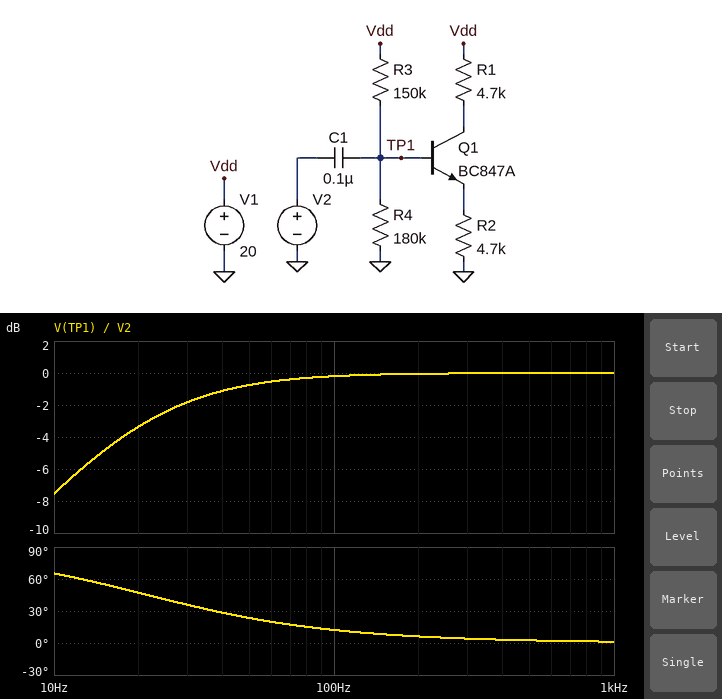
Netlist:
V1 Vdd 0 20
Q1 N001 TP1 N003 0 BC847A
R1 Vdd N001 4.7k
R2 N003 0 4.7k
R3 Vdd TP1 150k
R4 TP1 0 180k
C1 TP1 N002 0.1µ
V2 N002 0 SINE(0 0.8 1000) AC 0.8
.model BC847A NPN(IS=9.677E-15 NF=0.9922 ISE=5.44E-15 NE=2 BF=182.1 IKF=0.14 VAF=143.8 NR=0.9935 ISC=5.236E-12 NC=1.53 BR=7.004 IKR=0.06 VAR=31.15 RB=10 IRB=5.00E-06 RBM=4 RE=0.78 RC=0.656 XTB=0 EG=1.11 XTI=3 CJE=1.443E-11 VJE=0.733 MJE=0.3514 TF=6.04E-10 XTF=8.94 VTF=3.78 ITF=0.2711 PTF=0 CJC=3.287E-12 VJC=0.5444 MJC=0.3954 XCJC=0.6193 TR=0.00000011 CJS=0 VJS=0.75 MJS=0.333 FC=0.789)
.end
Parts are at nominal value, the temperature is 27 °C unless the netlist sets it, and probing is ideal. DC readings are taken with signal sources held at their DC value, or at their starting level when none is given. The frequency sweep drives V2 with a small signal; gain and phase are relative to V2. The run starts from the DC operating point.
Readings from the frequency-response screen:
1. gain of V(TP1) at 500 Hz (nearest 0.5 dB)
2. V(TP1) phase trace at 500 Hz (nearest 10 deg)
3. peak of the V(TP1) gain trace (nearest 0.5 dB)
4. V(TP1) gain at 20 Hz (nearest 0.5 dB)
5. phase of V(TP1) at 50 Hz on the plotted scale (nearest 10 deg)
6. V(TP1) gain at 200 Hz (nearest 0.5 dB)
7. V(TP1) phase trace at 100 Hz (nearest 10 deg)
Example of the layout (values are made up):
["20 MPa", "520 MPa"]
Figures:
["0 dB", "0 deg", "0 dB", "-3.5 dB", "20 deg", "0 dB", "10 deg"]
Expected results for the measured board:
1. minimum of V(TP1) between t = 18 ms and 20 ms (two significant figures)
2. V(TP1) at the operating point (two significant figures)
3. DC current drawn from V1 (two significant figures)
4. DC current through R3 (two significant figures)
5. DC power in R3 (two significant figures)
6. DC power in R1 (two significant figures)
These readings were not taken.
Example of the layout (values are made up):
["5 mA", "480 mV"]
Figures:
["9.1 V", "10 V", "2.0 mA", "67 µA", "670 µW", "18 mW"]
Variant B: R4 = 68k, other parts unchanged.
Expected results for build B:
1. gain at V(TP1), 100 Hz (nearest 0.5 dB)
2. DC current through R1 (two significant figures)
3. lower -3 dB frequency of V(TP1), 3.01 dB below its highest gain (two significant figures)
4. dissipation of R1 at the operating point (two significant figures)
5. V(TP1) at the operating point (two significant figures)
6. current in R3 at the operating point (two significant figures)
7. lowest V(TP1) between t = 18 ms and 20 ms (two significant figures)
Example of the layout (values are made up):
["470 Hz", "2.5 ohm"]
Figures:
["-0.5 dB", "1.1 mA", "36 Hz", "5.9 mW", "6.0 V", "94 µA", "5.2 V"]
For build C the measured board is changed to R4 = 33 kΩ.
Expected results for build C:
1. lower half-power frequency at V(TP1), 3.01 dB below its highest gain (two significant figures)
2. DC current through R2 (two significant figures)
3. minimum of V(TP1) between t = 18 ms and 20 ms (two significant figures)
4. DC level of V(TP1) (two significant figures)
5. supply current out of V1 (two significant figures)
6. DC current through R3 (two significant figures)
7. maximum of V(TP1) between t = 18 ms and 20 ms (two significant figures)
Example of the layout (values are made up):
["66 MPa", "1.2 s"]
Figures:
["61 Hz", "610 µA", "2.7 V", "3.5 V", "720 µA", "110 µA", "4.3 V"]
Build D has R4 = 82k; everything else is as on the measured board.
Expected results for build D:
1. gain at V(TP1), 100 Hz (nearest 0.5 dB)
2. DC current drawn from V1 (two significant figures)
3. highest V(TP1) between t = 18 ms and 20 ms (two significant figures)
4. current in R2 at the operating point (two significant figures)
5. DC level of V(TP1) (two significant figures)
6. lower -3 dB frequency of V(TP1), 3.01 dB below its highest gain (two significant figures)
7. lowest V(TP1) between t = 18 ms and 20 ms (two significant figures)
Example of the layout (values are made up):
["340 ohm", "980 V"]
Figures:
["-0.5 dB", "1.4 mA", "7.5 V", "1.3 mA", "6.7 V", "32 Hz", "5.9 V"]
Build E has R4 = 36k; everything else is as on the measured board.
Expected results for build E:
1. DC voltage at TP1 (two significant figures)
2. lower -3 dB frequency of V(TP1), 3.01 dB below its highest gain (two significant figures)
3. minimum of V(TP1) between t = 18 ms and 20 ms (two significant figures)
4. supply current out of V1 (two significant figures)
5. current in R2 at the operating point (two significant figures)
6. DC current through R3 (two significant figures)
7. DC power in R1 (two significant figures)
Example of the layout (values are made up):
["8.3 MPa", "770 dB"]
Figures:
["3.8 V", "57 Hz", "3.0 V", "770 µA", "670 µA", "110 µA", "2.1 mW"]
